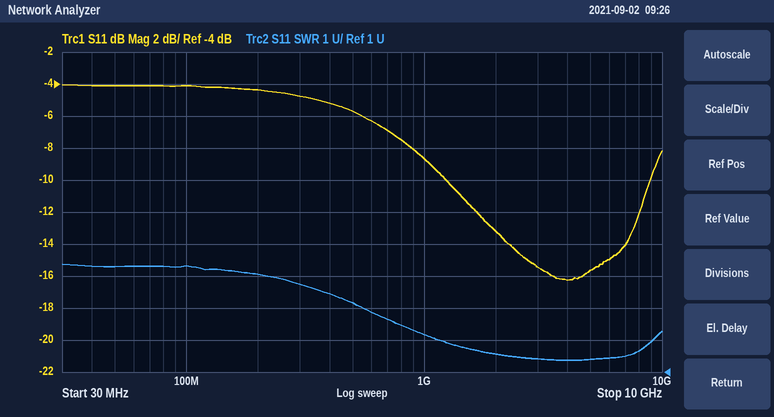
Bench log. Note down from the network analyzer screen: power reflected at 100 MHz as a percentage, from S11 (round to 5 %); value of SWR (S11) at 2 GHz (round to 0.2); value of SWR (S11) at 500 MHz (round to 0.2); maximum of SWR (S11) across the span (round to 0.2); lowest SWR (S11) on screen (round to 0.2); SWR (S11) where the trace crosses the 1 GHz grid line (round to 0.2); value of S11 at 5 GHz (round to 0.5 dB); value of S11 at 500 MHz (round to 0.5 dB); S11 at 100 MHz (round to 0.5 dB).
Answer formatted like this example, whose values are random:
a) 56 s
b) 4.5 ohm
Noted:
a) 40 %
b) 1.6
c) 3.2
d) 4.4
e) 1.4
f) 2.2
g) -15.5 dB
h) -5.5 dB
i) -4.0 dB
